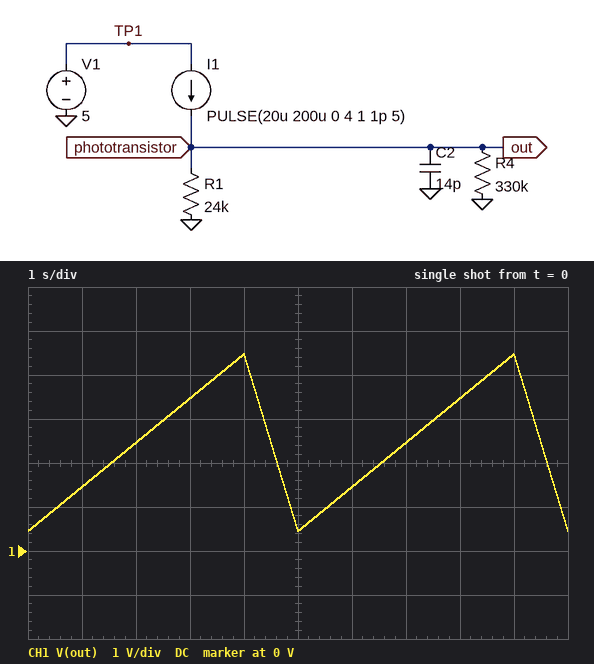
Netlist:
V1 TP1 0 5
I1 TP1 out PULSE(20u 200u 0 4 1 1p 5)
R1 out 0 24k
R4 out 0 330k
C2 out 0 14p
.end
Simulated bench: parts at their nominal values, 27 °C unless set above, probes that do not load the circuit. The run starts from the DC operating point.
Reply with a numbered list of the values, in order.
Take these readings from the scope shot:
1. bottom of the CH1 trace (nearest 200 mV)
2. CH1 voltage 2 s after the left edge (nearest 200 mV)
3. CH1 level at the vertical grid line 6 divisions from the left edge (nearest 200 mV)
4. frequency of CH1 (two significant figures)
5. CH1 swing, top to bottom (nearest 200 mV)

1. 400 mV
2. 2.4 V
3. 1.4 V
4. 200 mHz
5. 4.0 V
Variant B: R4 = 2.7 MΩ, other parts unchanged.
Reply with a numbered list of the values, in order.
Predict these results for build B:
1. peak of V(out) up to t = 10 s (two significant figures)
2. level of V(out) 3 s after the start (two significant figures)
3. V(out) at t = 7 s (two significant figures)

1. 4.8 V
2. 3.7 V
3. 2.6 V
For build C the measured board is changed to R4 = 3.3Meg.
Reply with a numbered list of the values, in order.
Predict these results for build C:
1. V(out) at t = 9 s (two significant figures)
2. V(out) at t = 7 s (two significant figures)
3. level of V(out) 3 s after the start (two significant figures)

1. 4.8 V
2. 2.6 V
3. 3.7 V
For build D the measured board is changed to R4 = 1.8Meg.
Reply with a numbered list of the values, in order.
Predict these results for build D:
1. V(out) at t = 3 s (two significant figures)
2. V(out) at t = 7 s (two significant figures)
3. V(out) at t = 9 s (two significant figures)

1. 3.7 V
2. 2.6 V
3. 4.7 V
